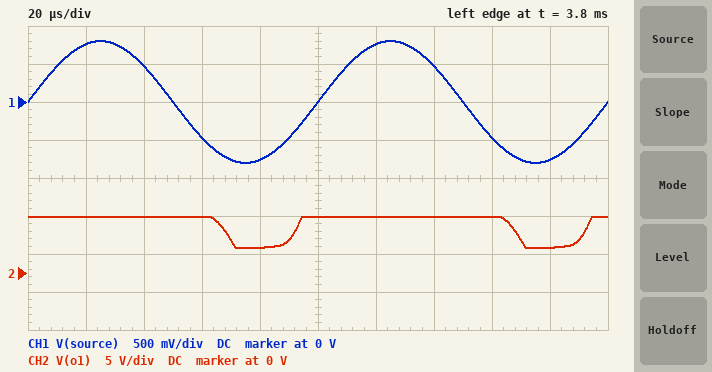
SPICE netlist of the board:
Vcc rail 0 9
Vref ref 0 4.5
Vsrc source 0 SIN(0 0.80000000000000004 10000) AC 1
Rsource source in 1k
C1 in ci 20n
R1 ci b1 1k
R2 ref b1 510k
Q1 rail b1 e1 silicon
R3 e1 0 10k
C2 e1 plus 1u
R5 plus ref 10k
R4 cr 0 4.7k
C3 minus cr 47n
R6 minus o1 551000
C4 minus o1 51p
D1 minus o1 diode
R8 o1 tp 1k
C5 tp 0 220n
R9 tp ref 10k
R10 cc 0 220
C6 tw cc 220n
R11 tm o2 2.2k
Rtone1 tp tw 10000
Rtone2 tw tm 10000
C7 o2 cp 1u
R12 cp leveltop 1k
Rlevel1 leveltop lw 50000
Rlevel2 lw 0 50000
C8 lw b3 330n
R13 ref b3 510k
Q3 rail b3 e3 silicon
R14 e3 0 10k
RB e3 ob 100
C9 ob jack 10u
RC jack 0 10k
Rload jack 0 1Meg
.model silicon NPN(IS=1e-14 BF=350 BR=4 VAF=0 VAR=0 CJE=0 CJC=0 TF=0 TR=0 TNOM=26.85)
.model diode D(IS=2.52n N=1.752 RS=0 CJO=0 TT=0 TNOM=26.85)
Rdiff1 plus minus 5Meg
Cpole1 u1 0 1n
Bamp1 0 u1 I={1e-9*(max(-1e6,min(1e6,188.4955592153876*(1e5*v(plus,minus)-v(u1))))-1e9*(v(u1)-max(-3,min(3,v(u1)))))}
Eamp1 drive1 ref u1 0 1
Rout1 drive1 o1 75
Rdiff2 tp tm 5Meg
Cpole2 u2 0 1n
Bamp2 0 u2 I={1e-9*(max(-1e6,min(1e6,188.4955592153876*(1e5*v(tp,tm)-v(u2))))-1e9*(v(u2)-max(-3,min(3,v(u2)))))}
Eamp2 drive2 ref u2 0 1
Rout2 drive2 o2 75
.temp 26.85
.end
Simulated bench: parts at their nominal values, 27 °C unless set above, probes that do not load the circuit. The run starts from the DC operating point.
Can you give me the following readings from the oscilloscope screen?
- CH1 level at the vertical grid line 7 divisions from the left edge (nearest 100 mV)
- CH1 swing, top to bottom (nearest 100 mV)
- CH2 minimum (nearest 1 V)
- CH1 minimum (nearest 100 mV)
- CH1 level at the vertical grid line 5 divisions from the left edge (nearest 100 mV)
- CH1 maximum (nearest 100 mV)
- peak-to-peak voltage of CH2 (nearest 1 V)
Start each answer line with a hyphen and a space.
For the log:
- 500 mV
- 1.6 V
- 3 V
- -800 mV
- 0 V
- 800 mV
- 4 V
